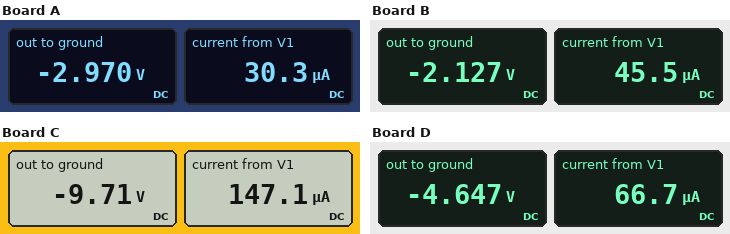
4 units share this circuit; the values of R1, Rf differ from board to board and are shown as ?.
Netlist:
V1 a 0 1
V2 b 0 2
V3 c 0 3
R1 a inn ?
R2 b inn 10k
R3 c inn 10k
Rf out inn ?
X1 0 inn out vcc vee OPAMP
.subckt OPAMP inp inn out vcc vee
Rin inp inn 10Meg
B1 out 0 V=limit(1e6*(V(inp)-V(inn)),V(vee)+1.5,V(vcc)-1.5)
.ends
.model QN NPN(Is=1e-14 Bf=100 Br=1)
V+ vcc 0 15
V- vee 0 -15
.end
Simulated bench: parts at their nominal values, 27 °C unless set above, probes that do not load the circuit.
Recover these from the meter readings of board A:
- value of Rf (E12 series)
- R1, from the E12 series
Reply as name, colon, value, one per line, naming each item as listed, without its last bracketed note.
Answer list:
value of Rf: 5.6 kΩ
R1, from the E12 series: 33 kΩ
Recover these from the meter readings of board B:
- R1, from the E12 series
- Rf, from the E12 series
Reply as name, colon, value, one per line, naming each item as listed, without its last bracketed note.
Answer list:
R1, from the E12 series: 22 kΩ
Rf, from the E12 series: 3.9 kΩ
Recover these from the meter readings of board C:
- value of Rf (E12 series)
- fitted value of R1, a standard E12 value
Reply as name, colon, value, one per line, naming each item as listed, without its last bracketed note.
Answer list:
value of Rf: 15 kΩ
fitted value of R1, a standard E12 value: 6.8 kΩ
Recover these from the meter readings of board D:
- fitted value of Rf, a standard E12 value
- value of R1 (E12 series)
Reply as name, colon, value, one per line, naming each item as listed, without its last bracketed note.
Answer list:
fitted value of Rf, a standard E12 value: 8.2 kΩ
value of R1: 15 kΩ
